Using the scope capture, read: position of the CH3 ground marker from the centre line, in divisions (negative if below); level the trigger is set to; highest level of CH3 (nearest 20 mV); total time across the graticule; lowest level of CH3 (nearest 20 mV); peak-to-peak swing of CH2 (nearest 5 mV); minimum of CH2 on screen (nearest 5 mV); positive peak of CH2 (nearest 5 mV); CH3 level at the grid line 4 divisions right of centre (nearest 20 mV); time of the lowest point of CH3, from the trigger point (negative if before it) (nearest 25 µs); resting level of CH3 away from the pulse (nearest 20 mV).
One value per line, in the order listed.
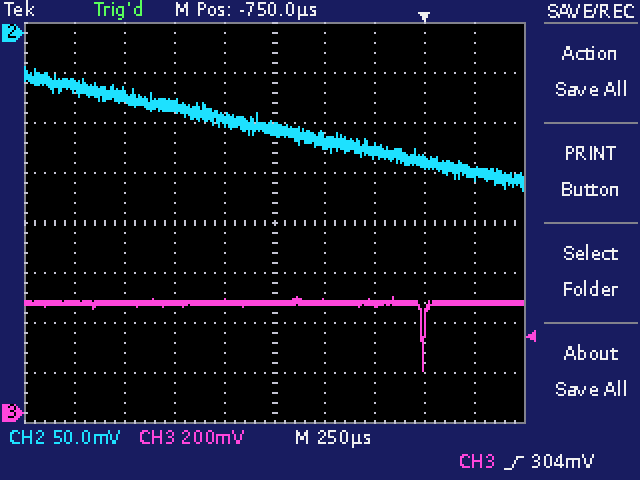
-3.8 div
304 mV
460 mV
2.5 ms
160 mV
125 mV
-160 mV
-35 mV
440 mV
0 µs
440 mV
